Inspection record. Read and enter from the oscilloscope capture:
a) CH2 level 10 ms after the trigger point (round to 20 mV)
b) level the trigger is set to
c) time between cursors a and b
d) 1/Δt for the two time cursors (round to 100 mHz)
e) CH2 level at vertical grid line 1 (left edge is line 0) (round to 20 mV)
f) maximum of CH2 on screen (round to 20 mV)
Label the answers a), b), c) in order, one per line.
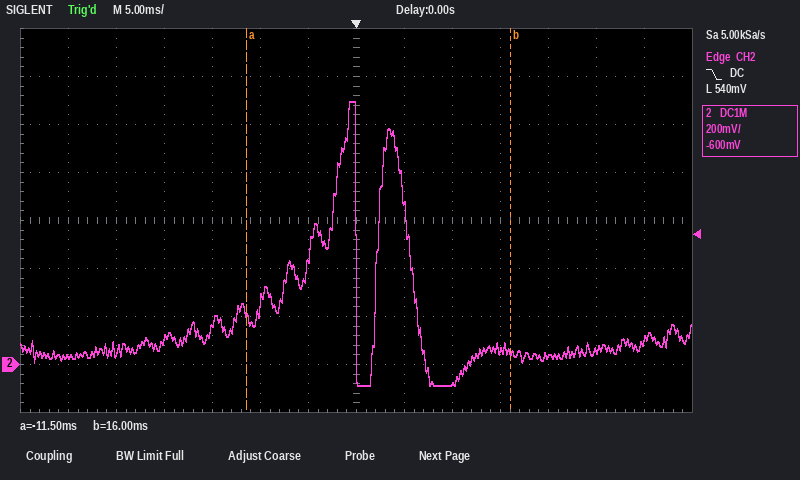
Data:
a) -80 mV
b) 540 mV
c) 27.5 ms
d) 36.4 Hz
e) 40 mV
f) 1.10 V
